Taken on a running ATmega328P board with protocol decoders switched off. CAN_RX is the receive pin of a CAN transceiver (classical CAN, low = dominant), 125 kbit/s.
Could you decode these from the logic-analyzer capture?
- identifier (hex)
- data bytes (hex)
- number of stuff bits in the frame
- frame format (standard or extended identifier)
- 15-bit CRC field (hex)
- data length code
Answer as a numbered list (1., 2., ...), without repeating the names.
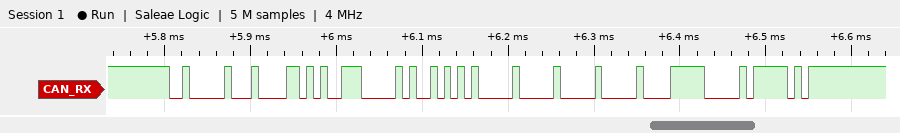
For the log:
1. 0x201
2. A7 02 55 00 00 00
3. 9
4. standard
5. 0x7C1F
6. 6
